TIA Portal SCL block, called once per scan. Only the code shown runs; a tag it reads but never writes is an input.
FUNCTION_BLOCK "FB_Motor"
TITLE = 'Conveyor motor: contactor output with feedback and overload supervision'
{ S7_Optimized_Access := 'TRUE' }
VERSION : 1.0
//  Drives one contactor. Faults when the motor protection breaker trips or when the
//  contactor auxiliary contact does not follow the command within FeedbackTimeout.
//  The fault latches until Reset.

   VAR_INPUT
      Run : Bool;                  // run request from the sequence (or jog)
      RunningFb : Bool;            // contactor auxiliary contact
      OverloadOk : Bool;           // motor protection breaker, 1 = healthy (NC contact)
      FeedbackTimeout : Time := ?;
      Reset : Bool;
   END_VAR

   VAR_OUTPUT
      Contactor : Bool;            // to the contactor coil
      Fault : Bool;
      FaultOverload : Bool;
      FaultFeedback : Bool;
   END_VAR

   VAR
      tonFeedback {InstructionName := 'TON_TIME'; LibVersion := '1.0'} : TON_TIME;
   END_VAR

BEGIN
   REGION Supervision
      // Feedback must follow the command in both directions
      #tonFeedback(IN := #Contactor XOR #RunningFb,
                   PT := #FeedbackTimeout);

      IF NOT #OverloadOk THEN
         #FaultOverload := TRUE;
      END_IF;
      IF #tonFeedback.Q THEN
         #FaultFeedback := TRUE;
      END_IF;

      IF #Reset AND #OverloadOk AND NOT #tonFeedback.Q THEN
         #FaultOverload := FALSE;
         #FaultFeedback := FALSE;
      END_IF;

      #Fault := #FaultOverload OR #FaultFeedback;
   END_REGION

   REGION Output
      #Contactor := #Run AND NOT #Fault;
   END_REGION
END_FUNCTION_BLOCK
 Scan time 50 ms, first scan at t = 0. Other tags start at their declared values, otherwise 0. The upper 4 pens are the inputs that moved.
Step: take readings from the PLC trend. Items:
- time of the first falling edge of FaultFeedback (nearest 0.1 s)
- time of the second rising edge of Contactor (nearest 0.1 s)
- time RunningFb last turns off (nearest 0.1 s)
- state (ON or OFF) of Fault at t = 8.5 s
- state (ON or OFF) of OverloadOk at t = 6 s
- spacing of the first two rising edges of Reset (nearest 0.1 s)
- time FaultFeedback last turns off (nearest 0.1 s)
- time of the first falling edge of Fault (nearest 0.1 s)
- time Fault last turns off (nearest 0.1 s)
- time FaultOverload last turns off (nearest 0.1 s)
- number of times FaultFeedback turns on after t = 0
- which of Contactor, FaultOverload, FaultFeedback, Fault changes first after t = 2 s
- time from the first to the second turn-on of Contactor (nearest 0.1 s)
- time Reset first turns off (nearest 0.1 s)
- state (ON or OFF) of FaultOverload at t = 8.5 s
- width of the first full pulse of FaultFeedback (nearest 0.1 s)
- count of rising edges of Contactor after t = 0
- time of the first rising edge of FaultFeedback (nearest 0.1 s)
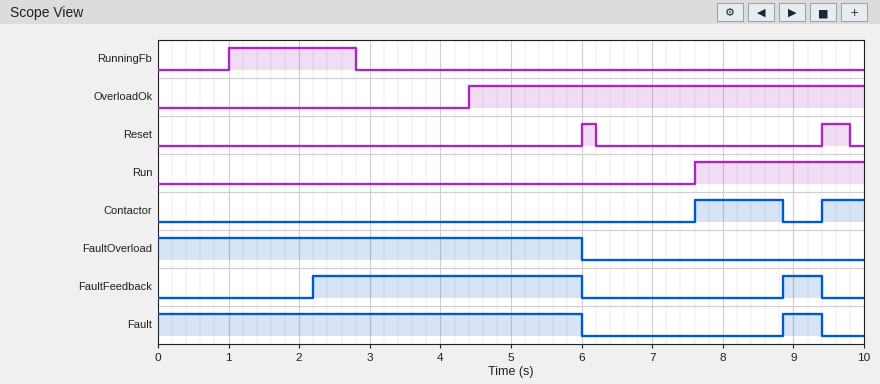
6.0 s
9.4 s
2.8 s
OFF
ON
3.4 s
9.4 s
6.0 s
9.4 s
6.0 s
2
FaultFeedback
1.8 s
6.2 s
OFF
3.8 s
2
2.2 s
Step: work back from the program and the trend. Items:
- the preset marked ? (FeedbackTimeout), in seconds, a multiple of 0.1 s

1.2 s
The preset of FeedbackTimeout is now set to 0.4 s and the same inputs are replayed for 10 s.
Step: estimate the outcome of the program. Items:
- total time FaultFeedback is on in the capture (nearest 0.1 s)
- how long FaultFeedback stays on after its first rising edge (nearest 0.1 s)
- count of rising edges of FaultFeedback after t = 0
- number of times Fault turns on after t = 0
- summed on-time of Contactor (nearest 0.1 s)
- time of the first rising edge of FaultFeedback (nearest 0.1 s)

6.1 s
4.6 s
3
2
0.9 s
1.4 s
